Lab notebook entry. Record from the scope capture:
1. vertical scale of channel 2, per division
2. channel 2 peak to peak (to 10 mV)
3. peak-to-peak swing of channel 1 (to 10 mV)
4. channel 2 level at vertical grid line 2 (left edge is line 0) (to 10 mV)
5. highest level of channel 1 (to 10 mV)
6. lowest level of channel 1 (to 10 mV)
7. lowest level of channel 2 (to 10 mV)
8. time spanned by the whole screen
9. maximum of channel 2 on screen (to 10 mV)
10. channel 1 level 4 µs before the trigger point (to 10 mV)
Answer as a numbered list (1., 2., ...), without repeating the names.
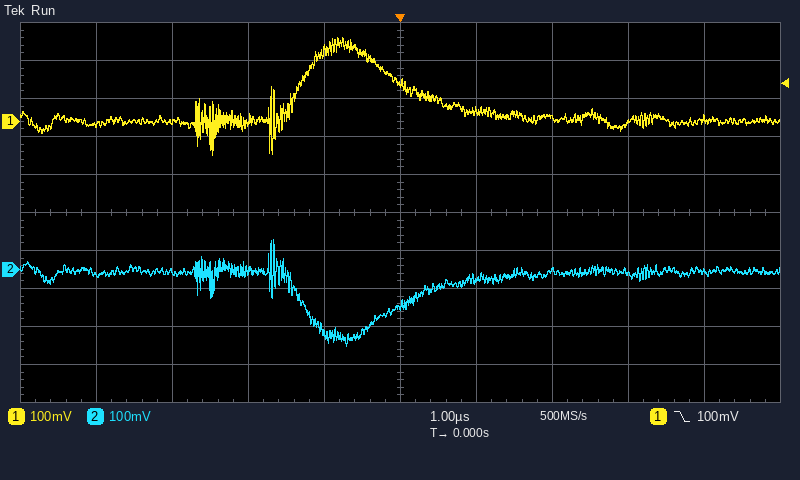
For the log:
1. 100 mV
2. 280 mV
3. 310 mV
4. -10 mV
5. 220 mV
6. -90 mV
7. -200 mV
8. 10 µs
9. 80 mV
10. -10 mV
